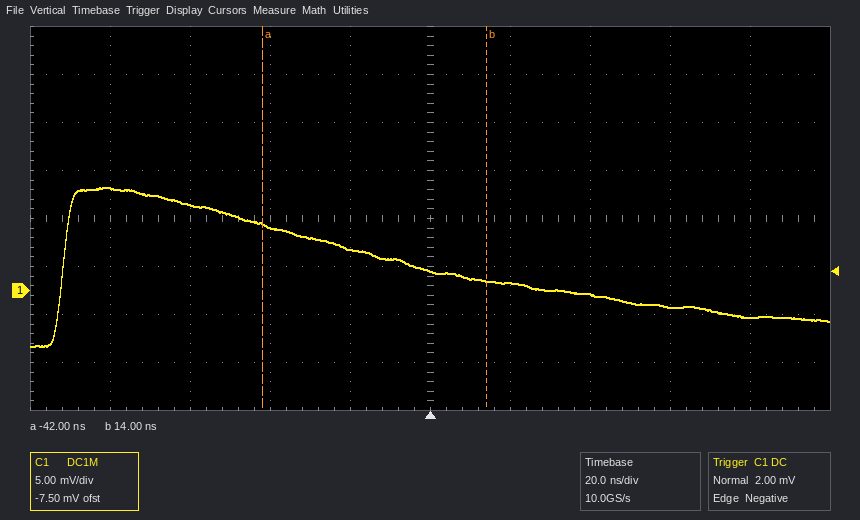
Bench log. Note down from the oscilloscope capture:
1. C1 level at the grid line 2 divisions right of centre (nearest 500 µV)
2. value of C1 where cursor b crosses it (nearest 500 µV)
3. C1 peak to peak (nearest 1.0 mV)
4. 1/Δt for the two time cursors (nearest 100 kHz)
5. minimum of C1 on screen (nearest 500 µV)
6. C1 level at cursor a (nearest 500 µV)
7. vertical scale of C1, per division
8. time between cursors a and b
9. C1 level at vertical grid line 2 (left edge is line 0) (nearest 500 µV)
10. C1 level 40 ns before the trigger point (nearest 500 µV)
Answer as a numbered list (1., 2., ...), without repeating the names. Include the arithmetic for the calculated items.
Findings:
1. -500 µV
2. 1.0 mV
3. 17.0 mV
4. 1 / 56 ns ≈ 17.9 MHz
5. -6.0 mV
6. 7.0 mV
7. 5 mV
8. 14 ns − (-42 ns) = 56 ns
9. 9.0 mV
10. 6.5 mV
